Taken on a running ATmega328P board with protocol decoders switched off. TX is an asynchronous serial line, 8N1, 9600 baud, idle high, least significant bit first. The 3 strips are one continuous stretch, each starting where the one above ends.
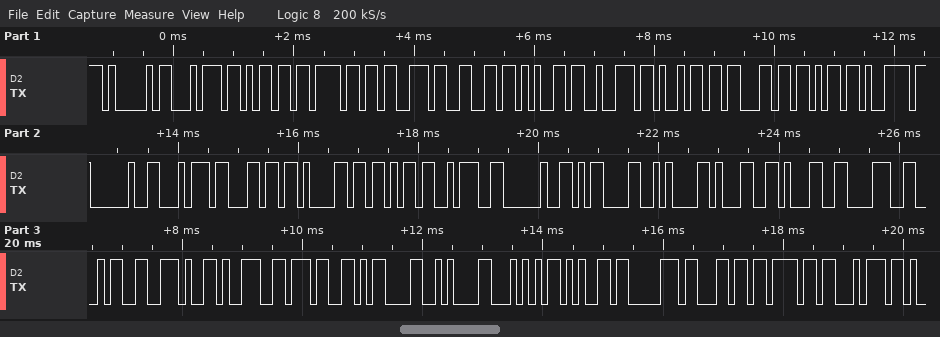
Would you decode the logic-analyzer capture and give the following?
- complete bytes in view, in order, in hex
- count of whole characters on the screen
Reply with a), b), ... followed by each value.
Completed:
a) 41 74 6D 6F 73 66 65 72 69 63 6B 79 20 74 6C 61 6B 3A 20 0D 0A 31 31 38 34 2E 39 37 0D 0A 54 65 70 6C 6F 74
b) 36
